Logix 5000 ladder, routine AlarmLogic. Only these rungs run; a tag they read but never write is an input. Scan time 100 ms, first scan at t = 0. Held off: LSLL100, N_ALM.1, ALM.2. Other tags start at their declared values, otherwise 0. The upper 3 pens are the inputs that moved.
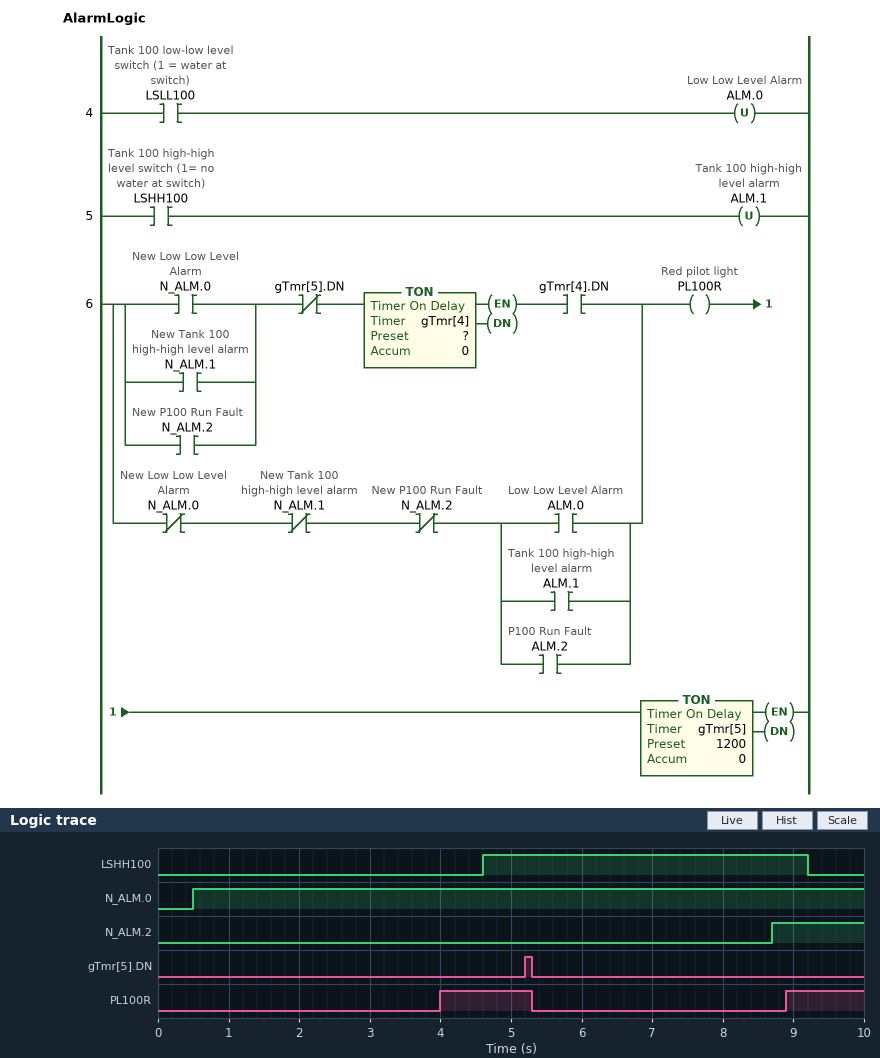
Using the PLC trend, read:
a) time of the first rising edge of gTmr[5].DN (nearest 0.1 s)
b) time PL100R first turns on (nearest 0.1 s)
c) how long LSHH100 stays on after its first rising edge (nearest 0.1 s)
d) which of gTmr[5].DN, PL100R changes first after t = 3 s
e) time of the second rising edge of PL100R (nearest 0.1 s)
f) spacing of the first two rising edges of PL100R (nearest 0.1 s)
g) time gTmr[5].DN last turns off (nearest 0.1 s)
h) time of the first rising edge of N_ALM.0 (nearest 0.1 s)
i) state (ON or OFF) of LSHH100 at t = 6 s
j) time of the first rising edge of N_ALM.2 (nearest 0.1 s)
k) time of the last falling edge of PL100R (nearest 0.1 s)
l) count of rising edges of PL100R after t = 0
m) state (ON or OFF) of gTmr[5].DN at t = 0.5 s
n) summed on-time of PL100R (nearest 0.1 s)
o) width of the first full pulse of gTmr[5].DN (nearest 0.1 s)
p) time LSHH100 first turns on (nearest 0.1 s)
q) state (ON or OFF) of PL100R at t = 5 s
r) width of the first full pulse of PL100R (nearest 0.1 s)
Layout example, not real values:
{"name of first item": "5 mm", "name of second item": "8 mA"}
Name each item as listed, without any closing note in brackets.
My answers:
{"time of the first rising edge of gTmr[5].DN": "5.2 s", "time PL100R first turns on": "4.0 s", "how long LSHH100 stays on after its first rising edge": "4.6 s", "which of gTmr[5].DN, PL100R changes first after t = 3 s": "PL100R", "time of the second rising edge of PL100R": "8.9 s", "spacing of the first two rising edges of PL100R": "4.9 s", "time gTmr[5].DN last turns off": "5.3 s", "time of the first rising edge of N_ALM.0": "0.5 s", "state (ON or OFF) of LSHH100 at t = 6 s": "ON", "time of the first rising edge of N_ALM.2": "8.7 s", "time of the last falling edge of PL100R": "5.3 s", "count of rising edges of PL100R after t = 0": "2", "state (ON or OFF) of gTmr[5].DN at t = 0.5 s": "OFF", "summed on-time of PL100R": "2.4 s", "width of the first full pulse of gTmr[5].DN": "0.1 s", "time LSHH100 first turns on": "4.6 s", "state (ON or OFF) of PL100R at t = 5 s": "ON", "width of the first full pulse of PL100R": "1.3 s"}
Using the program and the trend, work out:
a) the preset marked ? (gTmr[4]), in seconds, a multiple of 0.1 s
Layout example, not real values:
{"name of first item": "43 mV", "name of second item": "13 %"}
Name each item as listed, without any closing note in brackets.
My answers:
{"the preset marked ? (gTmr[4]), in seconds, a multiple of 0.1 s": "3.5 s"}
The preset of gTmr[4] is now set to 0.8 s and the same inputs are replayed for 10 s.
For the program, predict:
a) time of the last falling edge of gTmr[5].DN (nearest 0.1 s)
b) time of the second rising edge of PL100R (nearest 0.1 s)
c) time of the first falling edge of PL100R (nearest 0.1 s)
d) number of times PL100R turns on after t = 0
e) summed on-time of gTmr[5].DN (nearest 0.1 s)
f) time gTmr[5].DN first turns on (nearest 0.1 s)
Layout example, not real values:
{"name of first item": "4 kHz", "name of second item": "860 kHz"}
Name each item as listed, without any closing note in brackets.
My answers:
{"time of the last falling edge of gTmr[5].DN": "9.2 s", "time of the second rising edge of PL100R": "3.5 s", "time of the first falling edge of PL100R": "2.6 s", "number of times PL100R turns on after t = 0": "4", "summed on-time of gTmr[5].DN": "0.4 s", "time gTmr[5].DN first turns on": "2.5 s"}
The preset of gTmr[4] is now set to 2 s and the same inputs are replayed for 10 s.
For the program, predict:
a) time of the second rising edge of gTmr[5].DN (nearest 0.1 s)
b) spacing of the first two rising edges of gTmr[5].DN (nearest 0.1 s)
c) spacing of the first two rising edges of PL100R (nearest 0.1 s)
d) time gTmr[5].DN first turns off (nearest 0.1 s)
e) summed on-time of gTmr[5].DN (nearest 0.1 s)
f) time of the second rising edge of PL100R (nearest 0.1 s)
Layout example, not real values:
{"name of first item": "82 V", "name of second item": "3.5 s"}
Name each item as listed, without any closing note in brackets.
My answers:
{"time of the second rising edge of gTmr[5].DN": "7.1 s", "spacing of the first two rising edges of gTmr[5].DN": "3.4 s", "spacing of the first two rising edges of PL100R": "3.4 s", "time gTmr[5].DN first turns off": "3.8 s", "summed on-time of gTmr[5].DN": "0.2 s", "time of the second rising edge of PL100R": "5.9 s"}
